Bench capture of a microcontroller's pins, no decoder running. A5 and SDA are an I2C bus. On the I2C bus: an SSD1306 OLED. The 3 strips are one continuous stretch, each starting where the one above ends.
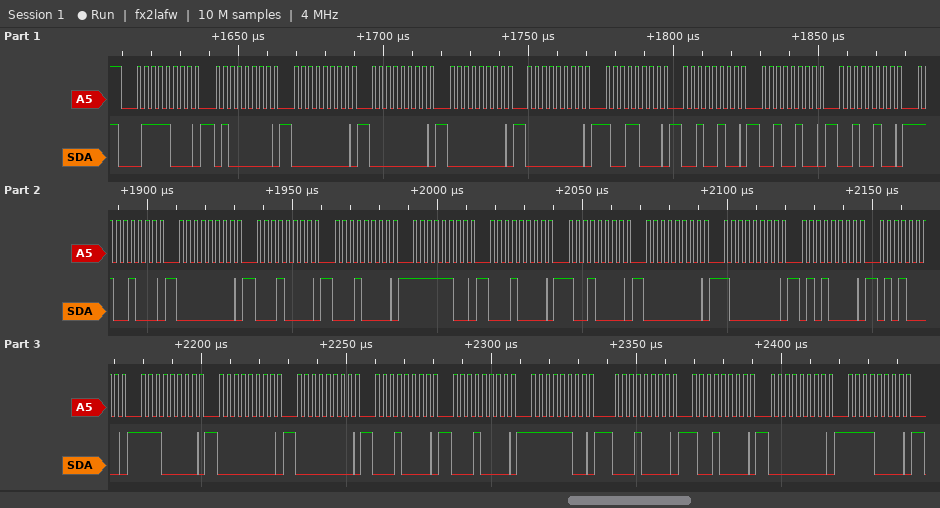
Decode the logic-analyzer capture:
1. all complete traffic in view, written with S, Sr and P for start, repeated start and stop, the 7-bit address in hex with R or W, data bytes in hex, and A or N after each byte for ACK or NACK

S 3CW A 40 A 00 A 00 A 00 A 00 A 98 A 24 A 24 A 24 A C8 A 00 A 10 A 10 A FC A 10 A 90 A 00 A 80 A 50 A 50 A E0 A 00 A 00 A 10 A 10 A FC A 10 A 90 A 00 A F0 A
